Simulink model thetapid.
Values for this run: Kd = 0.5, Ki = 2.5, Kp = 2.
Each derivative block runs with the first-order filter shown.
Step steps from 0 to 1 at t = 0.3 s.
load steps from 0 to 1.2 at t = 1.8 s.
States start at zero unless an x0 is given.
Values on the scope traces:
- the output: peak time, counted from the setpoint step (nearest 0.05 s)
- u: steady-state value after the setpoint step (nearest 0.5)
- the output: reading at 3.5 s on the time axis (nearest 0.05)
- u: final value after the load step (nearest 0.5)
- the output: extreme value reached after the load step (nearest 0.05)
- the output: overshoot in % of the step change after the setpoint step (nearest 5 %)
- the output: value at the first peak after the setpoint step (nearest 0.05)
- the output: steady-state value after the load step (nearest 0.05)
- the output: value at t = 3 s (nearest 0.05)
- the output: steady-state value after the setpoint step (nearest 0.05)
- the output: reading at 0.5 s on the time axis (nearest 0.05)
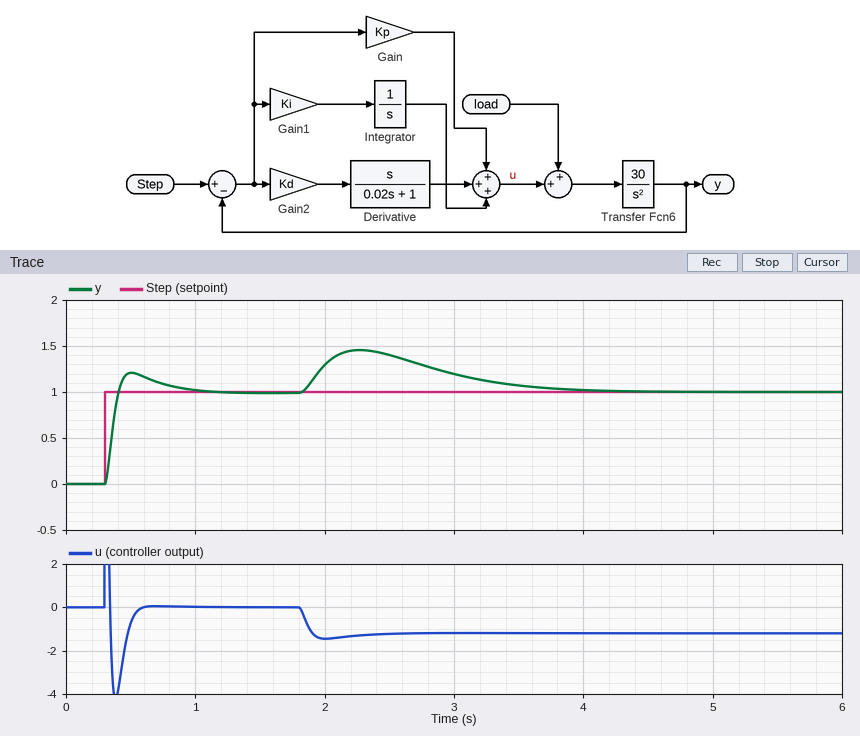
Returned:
0.20 s
0.0
1.05
-1.0
1.45
20 %
1.20
1.00
1.20
1.00
1.20
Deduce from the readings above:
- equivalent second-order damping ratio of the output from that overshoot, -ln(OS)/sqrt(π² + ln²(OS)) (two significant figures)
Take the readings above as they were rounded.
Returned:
0.46
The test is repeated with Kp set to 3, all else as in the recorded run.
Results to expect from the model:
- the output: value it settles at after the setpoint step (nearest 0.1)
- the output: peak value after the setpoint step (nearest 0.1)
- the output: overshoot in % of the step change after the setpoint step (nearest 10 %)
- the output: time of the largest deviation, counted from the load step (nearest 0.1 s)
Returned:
1.0
1.3
30 %
0.4 s
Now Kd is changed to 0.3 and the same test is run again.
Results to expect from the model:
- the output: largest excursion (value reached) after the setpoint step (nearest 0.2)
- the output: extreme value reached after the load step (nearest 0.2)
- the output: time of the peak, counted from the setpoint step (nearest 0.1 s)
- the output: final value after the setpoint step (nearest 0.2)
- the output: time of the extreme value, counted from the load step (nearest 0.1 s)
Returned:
1.4
1.6
0.3 s
1.0
0.4 s
